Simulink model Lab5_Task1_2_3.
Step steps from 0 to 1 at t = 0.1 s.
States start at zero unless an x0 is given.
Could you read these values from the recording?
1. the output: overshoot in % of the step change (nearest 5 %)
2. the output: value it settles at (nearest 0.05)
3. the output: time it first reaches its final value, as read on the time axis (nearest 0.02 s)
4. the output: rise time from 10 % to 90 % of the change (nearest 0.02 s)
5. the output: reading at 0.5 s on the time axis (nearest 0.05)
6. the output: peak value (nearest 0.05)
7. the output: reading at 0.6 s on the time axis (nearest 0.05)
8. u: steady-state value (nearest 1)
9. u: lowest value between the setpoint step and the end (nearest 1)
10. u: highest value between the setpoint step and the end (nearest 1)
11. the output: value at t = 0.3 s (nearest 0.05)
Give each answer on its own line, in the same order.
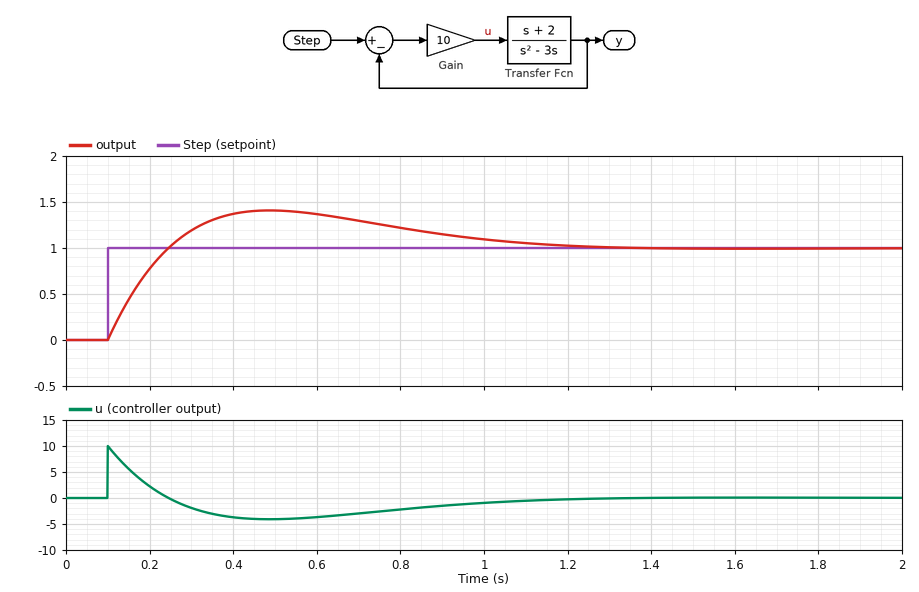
40 %
1.00
0.24 s
0.12 s
1.40
1.40
1.35
0
-4
10
1.20
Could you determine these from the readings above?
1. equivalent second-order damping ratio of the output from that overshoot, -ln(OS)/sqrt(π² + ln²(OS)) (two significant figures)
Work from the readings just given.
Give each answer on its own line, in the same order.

0.28
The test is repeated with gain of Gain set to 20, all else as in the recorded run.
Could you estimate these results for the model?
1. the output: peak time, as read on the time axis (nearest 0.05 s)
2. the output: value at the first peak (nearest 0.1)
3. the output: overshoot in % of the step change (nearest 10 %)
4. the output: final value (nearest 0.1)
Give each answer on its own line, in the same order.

0.35 s
1.2
20 %
1.0
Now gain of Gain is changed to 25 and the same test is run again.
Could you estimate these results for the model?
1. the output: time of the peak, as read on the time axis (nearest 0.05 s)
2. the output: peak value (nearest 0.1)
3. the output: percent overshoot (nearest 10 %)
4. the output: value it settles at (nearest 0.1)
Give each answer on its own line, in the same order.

0.30 s
1.2
20 %
1.0
